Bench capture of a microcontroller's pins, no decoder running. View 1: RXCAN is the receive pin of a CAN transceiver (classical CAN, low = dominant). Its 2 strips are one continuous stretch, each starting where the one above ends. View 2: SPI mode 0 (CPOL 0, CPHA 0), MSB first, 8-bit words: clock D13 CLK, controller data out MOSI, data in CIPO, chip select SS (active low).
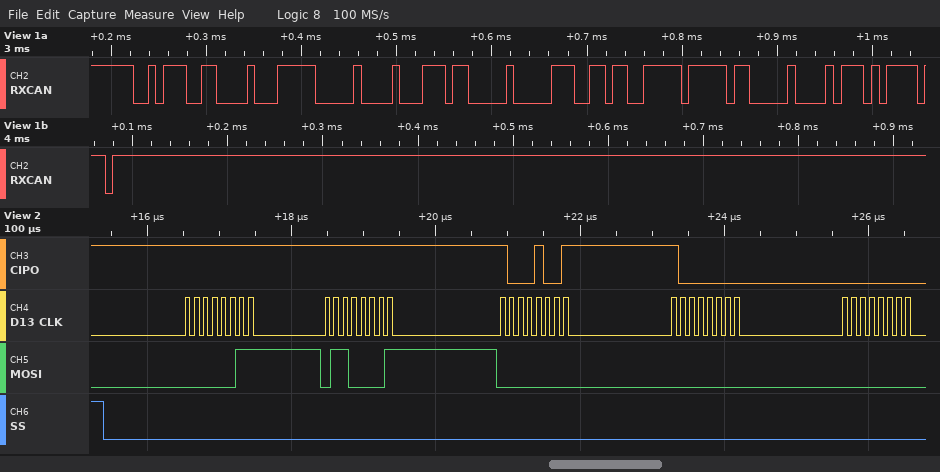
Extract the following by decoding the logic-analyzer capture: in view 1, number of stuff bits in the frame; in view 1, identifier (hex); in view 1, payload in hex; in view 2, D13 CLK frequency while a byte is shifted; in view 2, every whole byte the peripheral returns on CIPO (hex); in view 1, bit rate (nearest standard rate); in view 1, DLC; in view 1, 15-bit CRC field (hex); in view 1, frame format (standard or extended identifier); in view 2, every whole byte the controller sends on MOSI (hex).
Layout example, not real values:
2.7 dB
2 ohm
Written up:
7
0x2E6
F8 04 76 00 66 CF FF 00
8 MHz
FF FF 89 80 00
125 kbit/s
8
0x2EBD
standard
03 61 00 00 00
